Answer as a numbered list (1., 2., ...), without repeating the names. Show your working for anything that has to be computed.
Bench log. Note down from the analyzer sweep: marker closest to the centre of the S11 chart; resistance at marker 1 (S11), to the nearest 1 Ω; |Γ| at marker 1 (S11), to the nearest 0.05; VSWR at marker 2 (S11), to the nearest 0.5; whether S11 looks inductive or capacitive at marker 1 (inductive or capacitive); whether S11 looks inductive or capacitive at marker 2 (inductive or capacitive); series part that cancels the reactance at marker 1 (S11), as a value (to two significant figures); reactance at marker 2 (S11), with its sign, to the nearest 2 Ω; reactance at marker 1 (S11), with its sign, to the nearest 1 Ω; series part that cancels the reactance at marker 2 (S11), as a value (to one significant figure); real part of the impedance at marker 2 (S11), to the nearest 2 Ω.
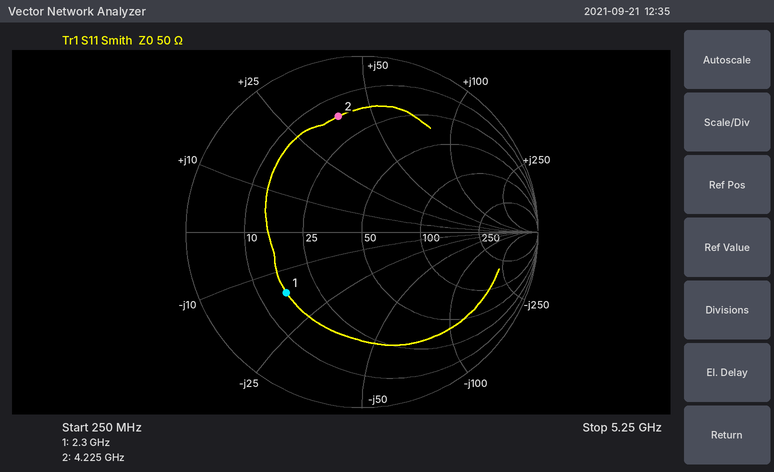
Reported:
1. marker 1
2. 16 Ω
3. 0.55
4. 5.0
5. capacitive
6. inductive
7. L = 16 Ω/(2π × 2.3 GHz) ≈ 1.1 nH
8. +38 Ω
9. -16 Ω
10. C = 1/(2π × 4.225 GHz × 38 Ω) ≈ 1.0 pF
11. 16 Ω
